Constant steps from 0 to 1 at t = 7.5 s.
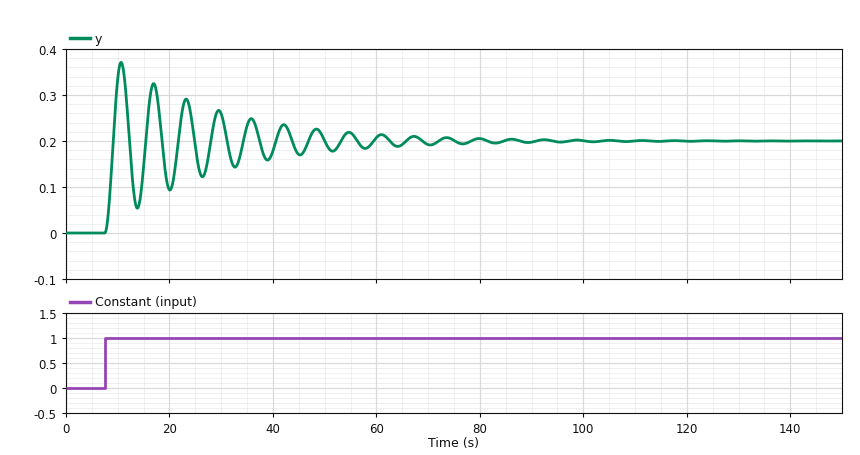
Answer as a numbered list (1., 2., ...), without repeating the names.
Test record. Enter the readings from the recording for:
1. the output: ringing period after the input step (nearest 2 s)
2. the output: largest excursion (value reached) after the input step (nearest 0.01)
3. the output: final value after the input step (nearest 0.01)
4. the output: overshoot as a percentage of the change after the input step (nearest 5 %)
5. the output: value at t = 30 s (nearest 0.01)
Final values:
1. 6 s
2. 0.37
3. 0.20
4. 85 %
5. 0.26
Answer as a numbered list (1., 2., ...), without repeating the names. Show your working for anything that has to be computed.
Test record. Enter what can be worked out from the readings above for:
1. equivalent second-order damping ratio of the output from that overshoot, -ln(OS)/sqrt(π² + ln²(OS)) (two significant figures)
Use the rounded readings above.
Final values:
1. ln(0.85) = -0.163; 0.163 / sqrt(9.870 + 0.026) = 0.052
